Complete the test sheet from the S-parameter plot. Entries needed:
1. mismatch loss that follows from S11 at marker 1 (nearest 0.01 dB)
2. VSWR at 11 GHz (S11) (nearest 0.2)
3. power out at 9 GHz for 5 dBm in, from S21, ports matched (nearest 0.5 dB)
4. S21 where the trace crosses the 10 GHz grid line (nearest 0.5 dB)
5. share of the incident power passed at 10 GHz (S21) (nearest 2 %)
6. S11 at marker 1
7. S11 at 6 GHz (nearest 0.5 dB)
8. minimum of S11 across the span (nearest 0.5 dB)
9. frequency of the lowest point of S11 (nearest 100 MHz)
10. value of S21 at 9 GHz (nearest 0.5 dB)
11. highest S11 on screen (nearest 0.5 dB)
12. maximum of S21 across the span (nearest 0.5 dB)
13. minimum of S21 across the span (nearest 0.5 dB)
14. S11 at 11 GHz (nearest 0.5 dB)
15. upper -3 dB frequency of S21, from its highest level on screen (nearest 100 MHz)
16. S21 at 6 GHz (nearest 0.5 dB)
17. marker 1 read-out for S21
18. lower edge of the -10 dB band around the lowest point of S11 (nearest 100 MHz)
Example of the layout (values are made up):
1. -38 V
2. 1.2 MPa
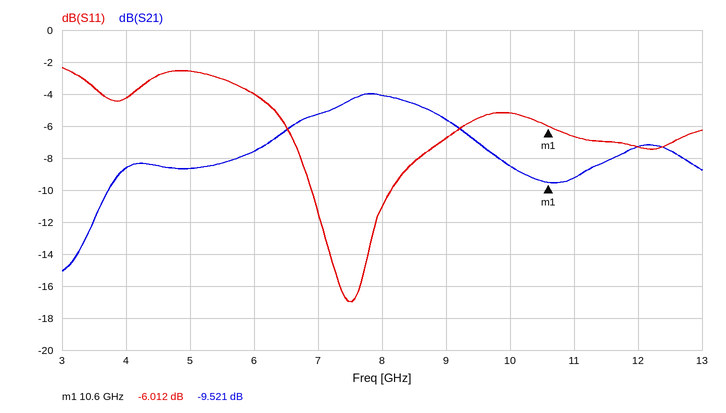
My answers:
1. 1.25 dB
2. 2.8
3. -0.5 dBm
4. -8.5 dB
5. 14 %
6. -6.012 dB
7. -4.0 dB
8. -17.0 dB
9. 7.5 GHz
10. -5.5 dB
11. -2.5 dB
12. -4.0 dB
13. -15.0 dB
14. -6.5 dB
15. 9.5 GHz
16. -7.5 dB
17. -9.521 dB
18. 6.9 GHz
